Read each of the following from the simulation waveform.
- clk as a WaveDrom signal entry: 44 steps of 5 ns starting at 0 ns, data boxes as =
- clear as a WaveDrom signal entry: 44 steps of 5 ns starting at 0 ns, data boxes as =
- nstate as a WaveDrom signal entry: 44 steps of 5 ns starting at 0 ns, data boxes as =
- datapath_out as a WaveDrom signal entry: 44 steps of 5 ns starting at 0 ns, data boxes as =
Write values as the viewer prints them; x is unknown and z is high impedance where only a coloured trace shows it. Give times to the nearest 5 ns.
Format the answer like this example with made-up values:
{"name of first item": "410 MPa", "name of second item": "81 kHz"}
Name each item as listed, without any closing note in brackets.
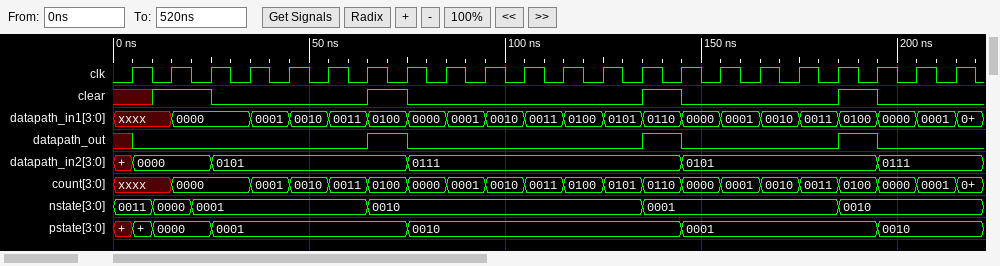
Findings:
{"clk as a WaveDrom signal entry: 44 steps of 5 ns starting at 0 ns, data boxes as =": "{name: 'clk', wave: '01010101010101010101010101010101010101010101'}", "clear as a WaveDrom signal entry: 44 steps of 5 ns starting at 0 ns, data boxes as =": "{name: 'clear', wave: 'x.1..0.......1.0...........1.0.......1.0....'}", "nstate as a WaveDrom signal entry: 44 steps of 5 ns starting at 0 ns, data boxes as =": "{name: 'nstate', wave: '=.=.=........=.............=.........=......', data: '0011 0000 0001 0010 0001 0010'}", "datapath_out as a WaveDrom signal entry: 44 steps of 5 ns starting at 0 ns, data boxes as =": "{name: 'datapath_out', wave: 'x0...........1.0...........1.0.......1.0....'}"}
